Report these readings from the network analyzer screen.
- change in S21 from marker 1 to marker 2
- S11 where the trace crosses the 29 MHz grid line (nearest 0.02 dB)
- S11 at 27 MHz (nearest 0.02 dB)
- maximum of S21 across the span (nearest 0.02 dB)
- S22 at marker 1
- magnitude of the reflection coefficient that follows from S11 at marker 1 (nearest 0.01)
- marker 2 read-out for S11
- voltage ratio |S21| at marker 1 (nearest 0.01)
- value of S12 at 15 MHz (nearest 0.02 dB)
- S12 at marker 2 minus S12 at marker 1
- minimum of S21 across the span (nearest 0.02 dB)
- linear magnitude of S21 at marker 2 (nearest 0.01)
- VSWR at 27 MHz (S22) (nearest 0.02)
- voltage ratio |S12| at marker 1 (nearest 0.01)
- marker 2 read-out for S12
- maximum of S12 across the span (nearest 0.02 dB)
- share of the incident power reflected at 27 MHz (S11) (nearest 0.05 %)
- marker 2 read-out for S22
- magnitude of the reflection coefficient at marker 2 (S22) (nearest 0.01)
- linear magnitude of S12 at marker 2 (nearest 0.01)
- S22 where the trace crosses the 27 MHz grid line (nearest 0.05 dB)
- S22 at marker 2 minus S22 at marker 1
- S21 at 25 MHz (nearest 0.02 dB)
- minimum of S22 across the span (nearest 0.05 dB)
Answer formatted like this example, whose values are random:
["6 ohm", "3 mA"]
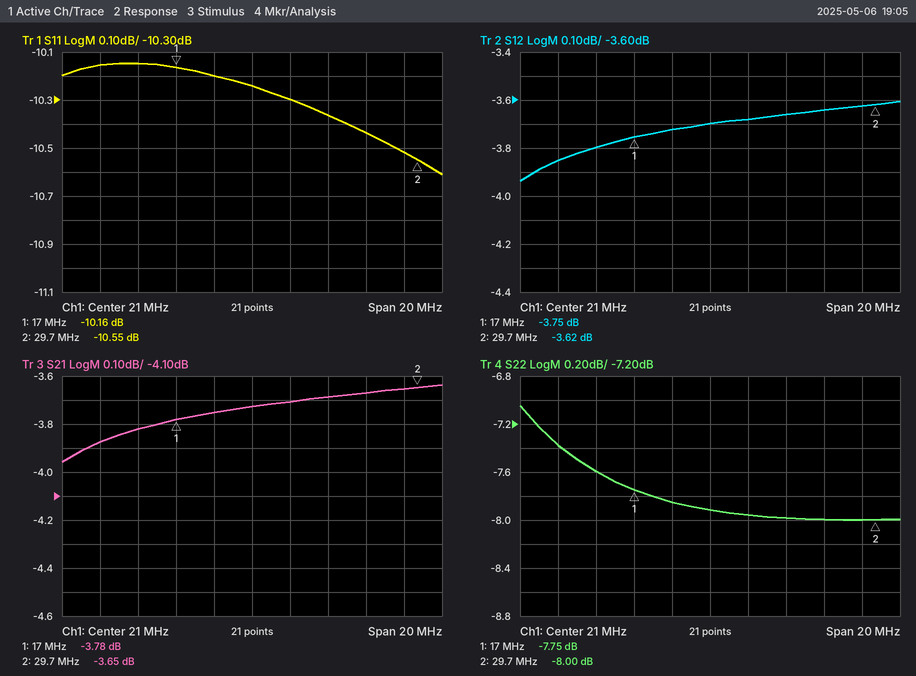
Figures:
["0.13 dB", "-10.52 dB", "-10.44 dB", "-3.64 dB", "-7.75 dB", "0.31", "-10.55 dB", "0.65", "-3.80 dB", "0.13 dB", "-3.96 dB", "0.66", "2.32", "0.65", "-3.62 dB", "-3.60 dB", "9.05 %", "-8.00 dB", "0.40", "0.66", "-8.00 dB", "-0.25 dB", "-3.68 dB", "-8.00 dB"]
